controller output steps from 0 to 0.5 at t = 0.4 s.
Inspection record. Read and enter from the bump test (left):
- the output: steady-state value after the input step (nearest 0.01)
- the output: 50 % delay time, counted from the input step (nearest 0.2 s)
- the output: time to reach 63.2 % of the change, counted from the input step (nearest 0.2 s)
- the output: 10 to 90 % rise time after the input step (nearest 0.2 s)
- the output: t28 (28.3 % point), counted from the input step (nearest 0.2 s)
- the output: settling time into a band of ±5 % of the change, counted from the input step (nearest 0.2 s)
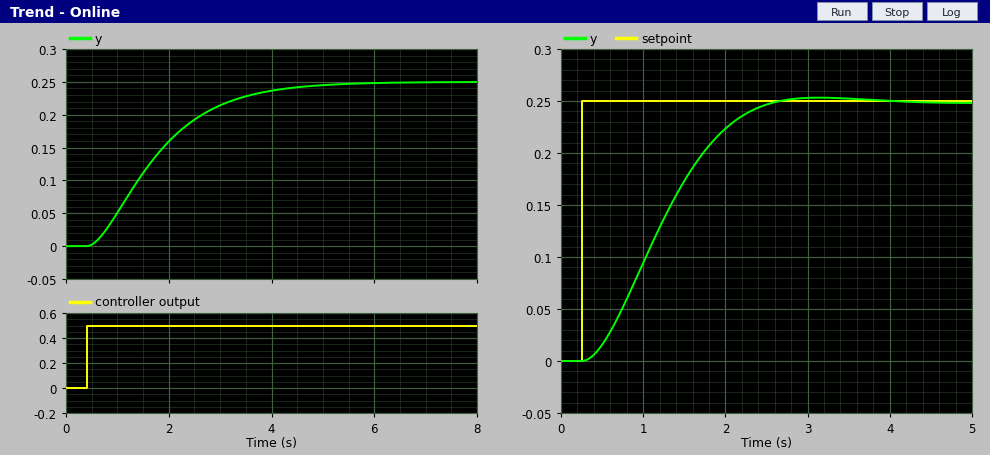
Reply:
0.25
1.2 s
1.6 s
2.6 s
0.8 s
3.6 s
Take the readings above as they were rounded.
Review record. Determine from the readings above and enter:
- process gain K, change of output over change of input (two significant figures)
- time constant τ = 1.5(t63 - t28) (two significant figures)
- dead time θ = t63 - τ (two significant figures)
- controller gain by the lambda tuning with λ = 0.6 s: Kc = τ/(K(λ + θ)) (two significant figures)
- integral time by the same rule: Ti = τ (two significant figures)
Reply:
0.50
1.2 s
0.40 s
2.4
1.2 s
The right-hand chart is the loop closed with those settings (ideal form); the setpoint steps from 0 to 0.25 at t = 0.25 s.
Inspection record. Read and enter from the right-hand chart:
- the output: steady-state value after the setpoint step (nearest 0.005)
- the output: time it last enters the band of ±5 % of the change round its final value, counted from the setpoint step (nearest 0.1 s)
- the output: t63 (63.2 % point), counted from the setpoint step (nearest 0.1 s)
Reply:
0.250
2.0 s
1.1 s
